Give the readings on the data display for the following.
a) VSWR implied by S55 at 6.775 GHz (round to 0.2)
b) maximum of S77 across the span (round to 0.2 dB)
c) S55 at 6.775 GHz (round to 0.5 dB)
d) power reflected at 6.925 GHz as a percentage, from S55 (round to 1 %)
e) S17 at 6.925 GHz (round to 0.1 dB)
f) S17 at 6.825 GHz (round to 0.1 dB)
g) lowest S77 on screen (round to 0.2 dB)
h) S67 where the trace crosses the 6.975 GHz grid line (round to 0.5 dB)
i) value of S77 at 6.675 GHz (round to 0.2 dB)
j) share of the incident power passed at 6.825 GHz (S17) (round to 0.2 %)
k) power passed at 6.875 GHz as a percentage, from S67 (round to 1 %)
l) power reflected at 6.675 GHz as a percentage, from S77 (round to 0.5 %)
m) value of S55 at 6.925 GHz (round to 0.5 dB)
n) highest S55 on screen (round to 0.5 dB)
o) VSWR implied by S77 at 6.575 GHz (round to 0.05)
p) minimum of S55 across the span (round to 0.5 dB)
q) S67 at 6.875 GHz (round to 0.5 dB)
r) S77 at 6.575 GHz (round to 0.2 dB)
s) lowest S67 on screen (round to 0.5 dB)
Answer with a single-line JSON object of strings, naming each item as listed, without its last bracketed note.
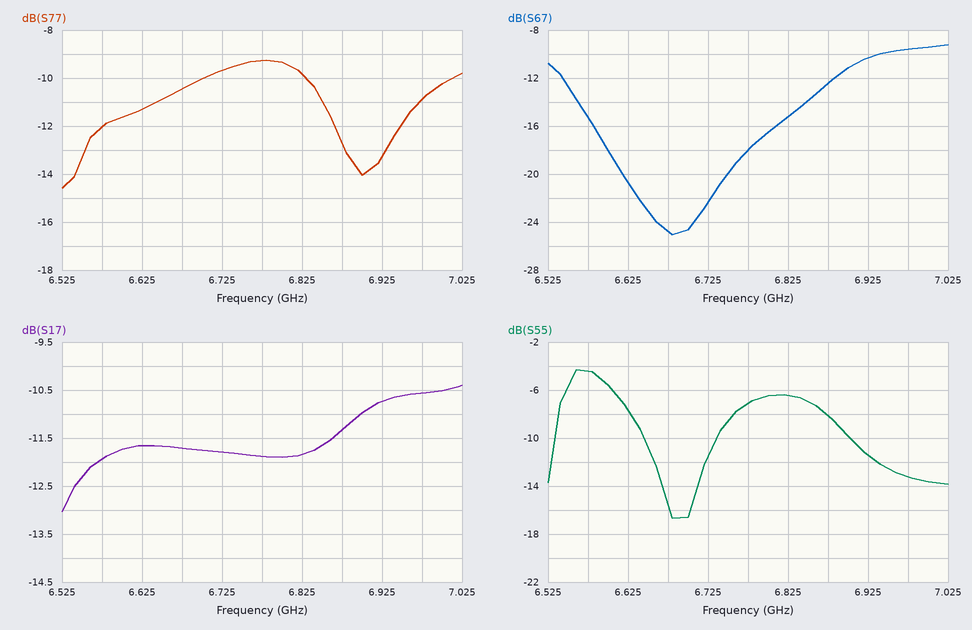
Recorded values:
{"VSWR implied by S55 at 6.775 GHz": "2.6", "maximum of S77 across the span": "-9.2 dB", "S55 at 6.775 GHz": "-7.0 dB", "power reflected at 6.925 GHz as a percentage, from S55": "7 %", "S17 at 6.925 GHz": "-10.7 dB", "S17 at 6.825 GHz": "-11.8 dB", "lowest S77 on screen": "-14.6 dB", "S67 where the trace crosses the 6.975 GHz grid line": "-9.5 dB", "value of S77 at 6.675 GHz": "-10.4 dB", "share of the incident power passed at 6.825 GHz (S17)": "6.6 %", "power passed at 6.875 GHz as a percentage, from S67": "6 %", "power reflected at 6.675 GHz as a percentage, from S77": "9.0 %", "value of S55 at 6.925 GHz": "-11.5 dB", "highest S55 on screen": "-4.5 dB", "VSWR implied by S77 at 6.575 GHz": "1.65", "minimum of S55 across the span": "-16.5 dB", "S67 at 6.875 GHz": "-12.5 dB", "S77 at 6.575 GHz": "-12.0 dB", "lowest S67 on screen": "-25.0 dB"}
